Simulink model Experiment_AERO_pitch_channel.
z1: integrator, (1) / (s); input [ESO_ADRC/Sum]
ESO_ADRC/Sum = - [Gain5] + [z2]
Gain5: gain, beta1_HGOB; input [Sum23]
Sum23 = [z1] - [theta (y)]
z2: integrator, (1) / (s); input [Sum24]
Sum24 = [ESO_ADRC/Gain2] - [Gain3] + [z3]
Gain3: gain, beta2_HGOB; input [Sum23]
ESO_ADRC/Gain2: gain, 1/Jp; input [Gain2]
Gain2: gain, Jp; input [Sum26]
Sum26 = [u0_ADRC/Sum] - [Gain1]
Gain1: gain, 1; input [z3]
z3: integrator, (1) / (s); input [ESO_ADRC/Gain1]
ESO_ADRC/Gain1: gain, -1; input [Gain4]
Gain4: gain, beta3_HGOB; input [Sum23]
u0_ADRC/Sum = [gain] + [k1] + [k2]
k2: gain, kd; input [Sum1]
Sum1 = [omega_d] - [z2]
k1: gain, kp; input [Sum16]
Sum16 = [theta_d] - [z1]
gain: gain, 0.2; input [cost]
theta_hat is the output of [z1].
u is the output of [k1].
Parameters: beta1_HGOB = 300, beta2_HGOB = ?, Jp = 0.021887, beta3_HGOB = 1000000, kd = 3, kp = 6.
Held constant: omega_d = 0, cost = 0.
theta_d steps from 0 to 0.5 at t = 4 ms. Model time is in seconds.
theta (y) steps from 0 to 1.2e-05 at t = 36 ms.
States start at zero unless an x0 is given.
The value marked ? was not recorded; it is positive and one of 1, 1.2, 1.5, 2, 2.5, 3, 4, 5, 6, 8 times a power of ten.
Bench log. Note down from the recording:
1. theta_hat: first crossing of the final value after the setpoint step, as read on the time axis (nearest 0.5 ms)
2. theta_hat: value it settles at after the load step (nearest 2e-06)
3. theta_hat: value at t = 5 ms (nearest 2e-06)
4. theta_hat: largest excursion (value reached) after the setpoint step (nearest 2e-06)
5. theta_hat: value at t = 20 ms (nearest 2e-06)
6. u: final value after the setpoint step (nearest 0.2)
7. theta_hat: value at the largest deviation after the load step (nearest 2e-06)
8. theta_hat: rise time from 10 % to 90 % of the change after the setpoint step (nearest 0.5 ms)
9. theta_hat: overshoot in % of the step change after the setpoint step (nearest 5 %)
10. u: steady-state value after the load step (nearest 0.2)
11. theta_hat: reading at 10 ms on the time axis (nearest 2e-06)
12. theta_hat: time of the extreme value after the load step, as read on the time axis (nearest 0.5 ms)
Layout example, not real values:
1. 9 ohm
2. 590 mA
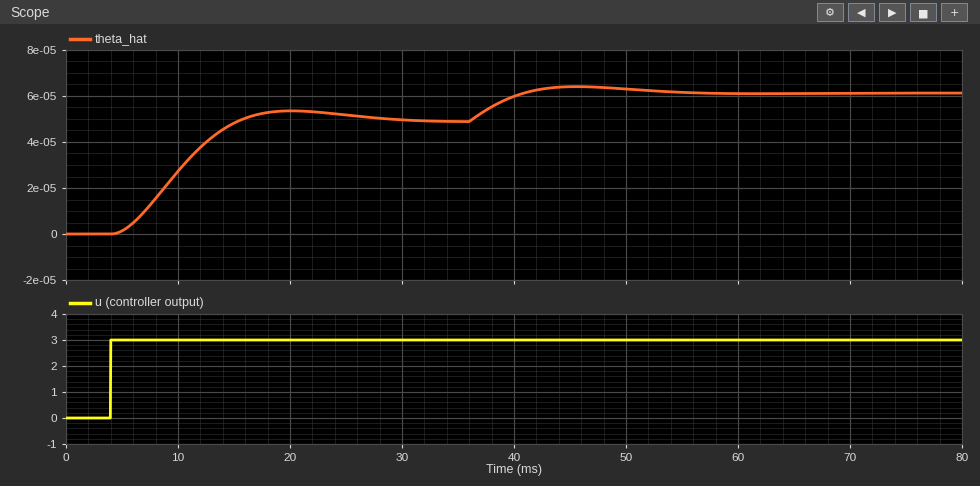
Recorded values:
1. 15.5 ms
2. 0.000062
3. 0.000002
4. 0.000054
5. 0.000054
6. 3.0
7. 0.000064
8. 7.5 ms
9. 10 %
10. 3.0
11. 0.000028
12. 45.5 ms
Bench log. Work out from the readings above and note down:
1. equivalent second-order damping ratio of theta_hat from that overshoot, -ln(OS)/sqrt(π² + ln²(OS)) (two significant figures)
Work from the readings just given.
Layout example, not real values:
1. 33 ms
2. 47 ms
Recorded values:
1. 0.59
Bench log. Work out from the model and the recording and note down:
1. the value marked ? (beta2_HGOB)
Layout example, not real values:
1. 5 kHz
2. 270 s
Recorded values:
1. 60000
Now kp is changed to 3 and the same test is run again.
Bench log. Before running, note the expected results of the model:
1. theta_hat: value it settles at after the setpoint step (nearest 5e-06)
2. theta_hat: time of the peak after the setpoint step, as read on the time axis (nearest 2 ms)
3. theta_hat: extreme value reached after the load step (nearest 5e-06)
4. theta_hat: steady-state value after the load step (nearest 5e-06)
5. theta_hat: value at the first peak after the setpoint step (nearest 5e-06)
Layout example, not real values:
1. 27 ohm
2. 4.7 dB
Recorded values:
1. 0.000025
2. 20 ms
3. 0.000040
4. 0.000035
5. 0.000025
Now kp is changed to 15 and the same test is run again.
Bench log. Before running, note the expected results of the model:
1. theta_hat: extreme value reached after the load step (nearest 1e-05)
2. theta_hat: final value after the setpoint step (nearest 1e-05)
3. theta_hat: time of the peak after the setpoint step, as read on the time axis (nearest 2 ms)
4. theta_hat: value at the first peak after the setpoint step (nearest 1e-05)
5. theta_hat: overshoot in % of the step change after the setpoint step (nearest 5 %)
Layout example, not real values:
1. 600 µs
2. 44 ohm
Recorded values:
1. 0.00014
2. 0.00012
3. 20 ms
4. 0.00013
5. 10 %
